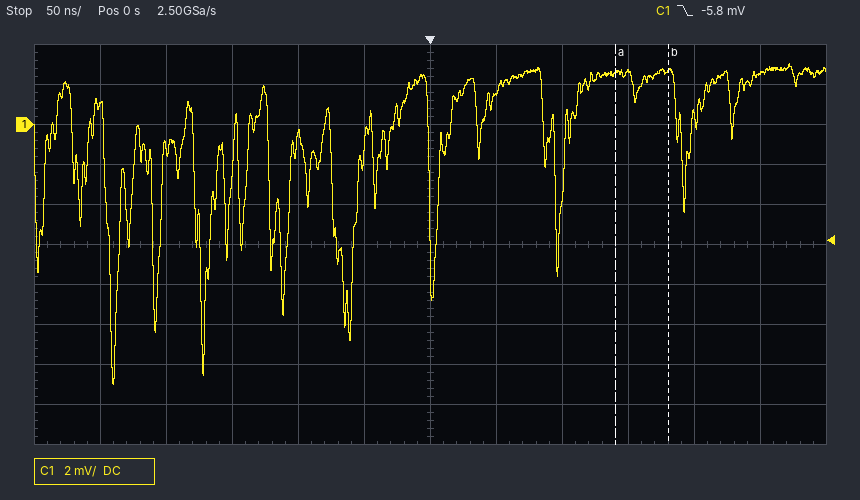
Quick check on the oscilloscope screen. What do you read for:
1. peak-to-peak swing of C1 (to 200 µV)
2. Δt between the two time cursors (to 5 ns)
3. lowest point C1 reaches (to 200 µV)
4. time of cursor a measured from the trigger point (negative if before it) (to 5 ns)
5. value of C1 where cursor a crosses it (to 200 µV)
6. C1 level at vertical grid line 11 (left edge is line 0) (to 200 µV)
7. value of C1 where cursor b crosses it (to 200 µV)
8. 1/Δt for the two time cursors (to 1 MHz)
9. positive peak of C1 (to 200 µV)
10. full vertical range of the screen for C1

16.0 mV
40 ns
-13.0 mV
+140 ns
2.6 mV
2.6 mV
2.6 mV
25 MHz
3.0 mV
20 mV
